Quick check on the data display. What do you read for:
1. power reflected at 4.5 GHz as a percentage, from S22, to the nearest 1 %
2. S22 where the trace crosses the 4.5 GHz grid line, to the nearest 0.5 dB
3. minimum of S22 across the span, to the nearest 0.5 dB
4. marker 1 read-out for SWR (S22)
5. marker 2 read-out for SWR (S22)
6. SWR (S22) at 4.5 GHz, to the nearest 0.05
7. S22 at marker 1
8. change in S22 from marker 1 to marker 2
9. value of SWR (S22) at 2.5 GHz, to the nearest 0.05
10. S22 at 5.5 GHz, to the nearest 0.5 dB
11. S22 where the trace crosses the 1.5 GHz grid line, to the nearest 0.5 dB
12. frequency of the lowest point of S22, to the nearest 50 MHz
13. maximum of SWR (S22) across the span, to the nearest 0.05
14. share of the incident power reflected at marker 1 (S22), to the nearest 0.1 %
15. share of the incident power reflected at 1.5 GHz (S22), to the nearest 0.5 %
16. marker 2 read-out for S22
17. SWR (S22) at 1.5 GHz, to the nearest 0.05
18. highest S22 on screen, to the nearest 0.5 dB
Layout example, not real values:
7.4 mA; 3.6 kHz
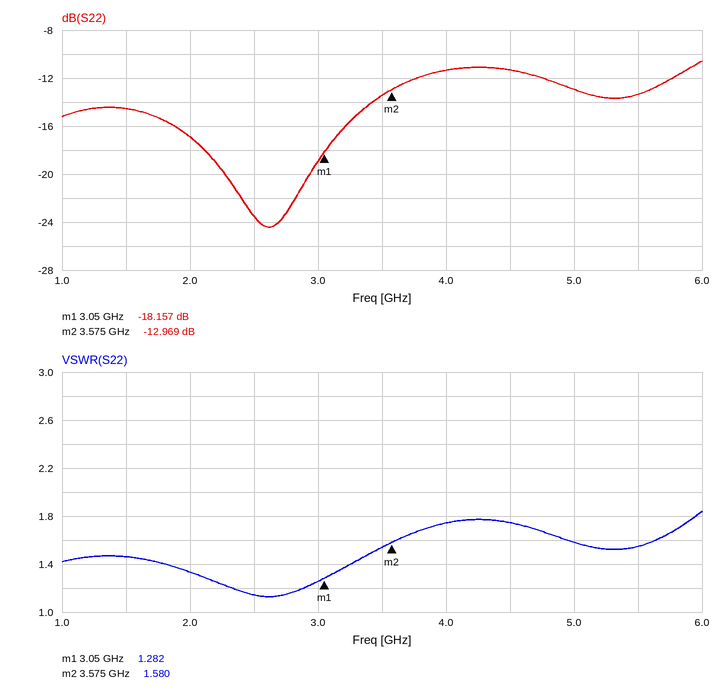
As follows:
7 %; -11.5 dB; -24.5 dB; 1.282; 1.580; 1.75; -18.157 dB; 5.188 dB; 1.15; -13.5 dB; -14.5 dB; 2.60 GHz; 1.85; 1.5 %; 3.5 %; -12.969 dB; 1.45; -10.5 dB
